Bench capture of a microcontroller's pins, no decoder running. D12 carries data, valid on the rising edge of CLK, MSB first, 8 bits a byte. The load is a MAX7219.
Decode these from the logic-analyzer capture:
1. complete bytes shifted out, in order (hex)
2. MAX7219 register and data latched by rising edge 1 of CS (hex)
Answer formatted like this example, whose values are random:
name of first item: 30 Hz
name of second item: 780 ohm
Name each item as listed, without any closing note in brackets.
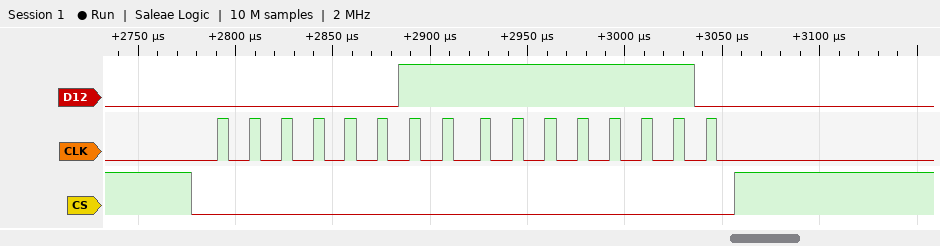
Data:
complete bytes shifted out, in order: 03 FE
MAX7219 register and data latched by rising edge 1 of CS: register 0x3, data 0xFE
